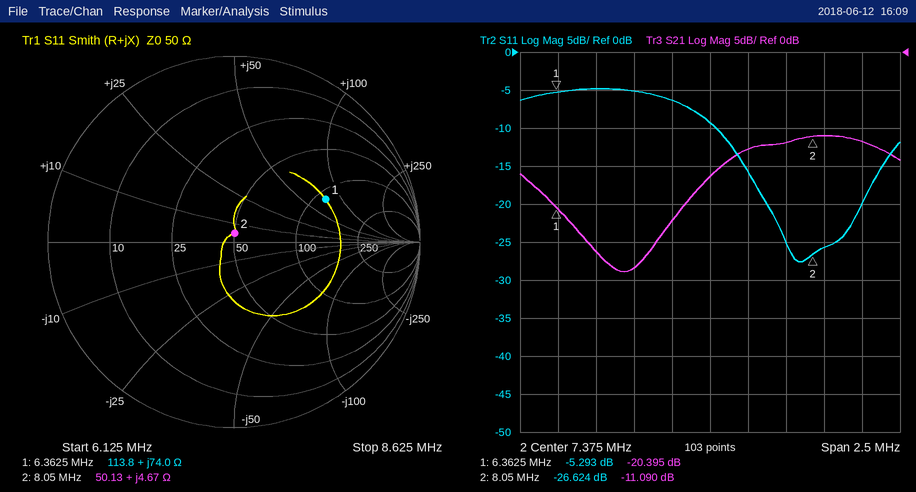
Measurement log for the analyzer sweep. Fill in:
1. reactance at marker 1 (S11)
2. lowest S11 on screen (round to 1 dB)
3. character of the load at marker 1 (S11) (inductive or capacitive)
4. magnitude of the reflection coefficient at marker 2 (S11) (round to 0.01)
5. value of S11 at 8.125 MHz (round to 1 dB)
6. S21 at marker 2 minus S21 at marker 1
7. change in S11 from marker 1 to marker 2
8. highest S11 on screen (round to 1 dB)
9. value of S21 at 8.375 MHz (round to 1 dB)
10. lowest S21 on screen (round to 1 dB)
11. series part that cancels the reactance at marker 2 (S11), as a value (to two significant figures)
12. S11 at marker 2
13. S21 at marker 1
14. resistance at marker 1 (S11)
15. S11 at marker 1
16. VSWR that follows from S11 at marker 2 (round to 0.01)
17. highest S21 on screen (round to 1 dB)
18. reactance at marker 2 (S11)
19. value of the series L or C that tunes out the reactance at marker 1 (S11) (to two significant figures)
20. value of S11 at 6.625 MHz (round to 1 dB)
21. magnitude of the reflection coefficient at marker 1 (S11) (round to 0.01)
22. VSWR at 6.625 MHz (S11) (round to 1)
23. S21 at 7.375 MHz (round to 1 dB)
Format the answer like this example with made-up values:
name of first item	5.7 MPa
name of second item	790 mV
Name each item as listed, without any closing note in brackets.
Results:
reactance at marker 1	+74.0 Ω
lowest S11 on screen	-28 dB
character of the load at marker 1 (S11)	inductive
magnitude of the reflection coefficient at marker 2 (S11)	0.05
value of S11 at 8.125 MHz	-26 dB
S21 at marker 2 minus S21 at marker 1	9.305 dB
change in S11 from marker 1 to marker 2	-21.331 dB
highest S11 on screen	-5 dB
value of S21 at 8.375 MHz	-12 dB
lowest S21 on screen	-29 dB
series part that cancels the reactance at marker 2 (S11), as a value	4.2 nF
S11 at marker 2	-26.624 dB
S21 at marker 1	-20.395 dB
resistance at marker 1	113.8 Ω
S11 at marker 1	-5.293 dB
VSWR that follows from S11 at marker 2	1.10
highest S21 on screen	-11 dB
reactance at marker 2	+4.67 Ω
value of the series L or C that tunes out the reactance at marker 1 (S11)	340 pF
value of S11 at 6.625 MHz	-5 dB
magnitude of the reflection coefficient at marker 1 (S11)	0.54
VSWR at 6.625 MHz (S11)	4
S21 at 7.375 MHz	-16 dB
